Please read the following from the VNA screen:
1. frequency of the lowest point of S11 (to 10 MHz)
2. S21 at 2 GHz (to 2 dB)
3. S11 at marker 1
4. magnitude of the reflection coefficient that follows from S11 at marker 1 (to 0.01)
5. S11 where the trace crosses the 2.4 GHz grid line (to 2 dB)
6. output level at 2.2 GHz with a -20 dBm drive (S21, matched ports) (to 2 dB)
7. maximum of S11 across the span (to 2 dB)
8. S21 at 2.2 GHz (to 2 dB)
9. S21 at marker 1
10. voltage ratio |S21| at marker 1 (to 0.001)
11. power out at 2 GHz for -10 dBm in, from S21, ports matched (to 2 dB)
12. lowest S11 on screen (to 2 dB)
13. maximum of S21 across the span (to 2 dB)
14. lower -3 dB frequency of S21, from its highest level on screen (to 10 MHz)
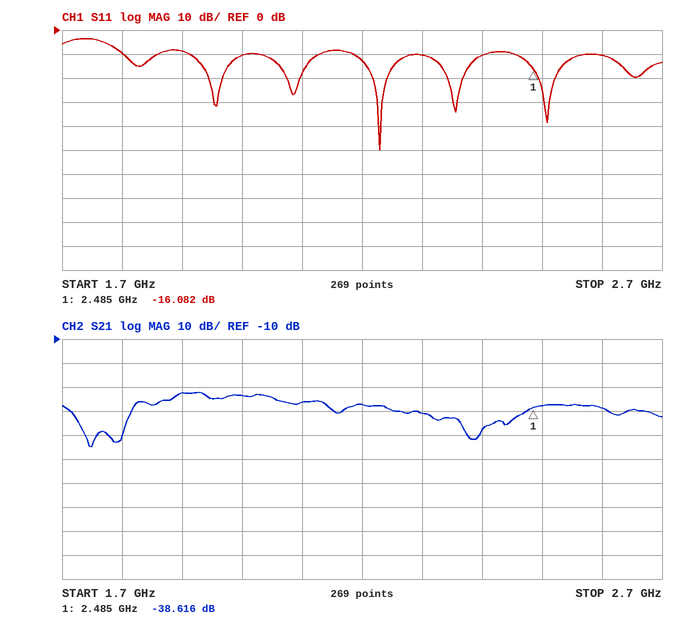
2.23 GHz
-34 dB
-16.082 dB
0.16
-10 dB
-58 dBm
-4 dB
-38 dB
-38.616 dB
0.012
-44 dBm
-50 dB
-32 dB
1.88 GHz
